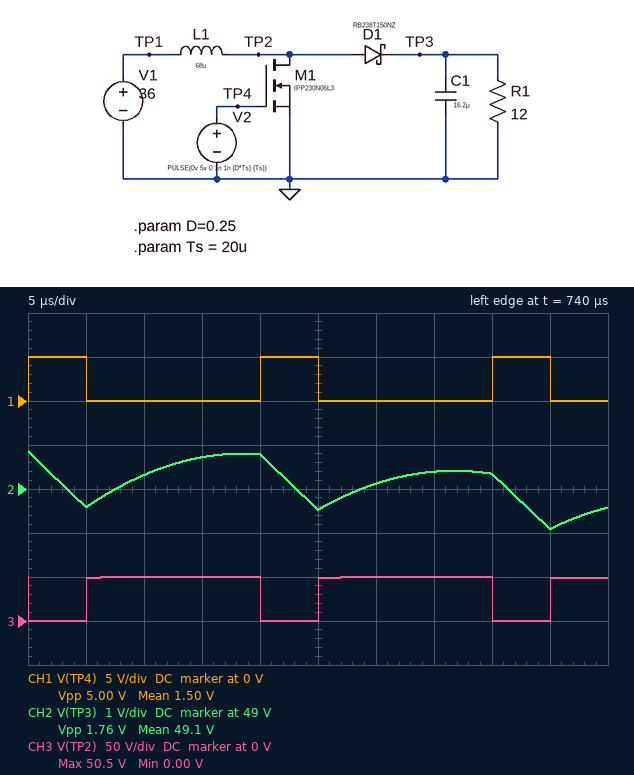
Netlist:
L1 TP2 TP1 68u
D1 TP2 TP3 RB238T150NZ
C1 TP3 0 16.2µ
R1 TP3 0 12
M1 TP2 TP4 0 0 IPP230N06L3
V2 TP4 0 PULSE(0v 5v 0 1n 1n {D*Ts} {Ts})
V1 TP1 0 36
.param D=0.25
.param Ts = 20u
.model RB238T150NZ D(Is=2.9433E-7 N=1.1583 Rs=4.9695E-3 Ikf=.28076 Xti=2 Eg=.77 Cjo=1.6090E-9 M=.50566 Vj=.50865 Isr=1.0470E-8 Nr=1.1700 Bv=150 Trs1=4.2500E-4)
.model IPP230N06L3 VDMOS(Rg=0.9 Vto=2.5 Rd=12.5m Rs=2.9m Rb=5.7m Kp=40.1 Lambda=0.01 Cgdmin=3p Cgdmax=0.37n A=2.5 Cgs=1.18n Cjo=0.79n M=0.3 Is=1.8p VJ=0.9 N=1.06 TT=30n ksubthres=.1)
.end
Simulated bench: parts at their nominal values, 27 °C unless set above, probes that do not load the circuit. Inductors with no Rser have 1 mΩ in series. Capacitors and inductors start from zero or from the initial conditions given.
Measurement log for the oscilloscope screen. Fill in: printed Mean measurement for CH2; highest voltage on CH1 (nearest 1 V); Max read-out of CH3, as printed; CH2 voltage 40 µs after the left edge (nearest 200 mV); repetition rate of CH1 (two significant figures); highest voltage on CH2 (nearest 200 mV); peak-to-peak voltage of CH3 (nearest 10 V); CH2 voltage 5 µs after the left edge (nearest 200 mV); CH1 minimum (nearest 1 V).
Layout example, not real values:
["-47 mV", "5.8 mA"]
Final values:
["49.1 V", "5 V", "50.5 V", "49.4 V", "50 kHz", "49.8 V", "50 V", "48.6 V", "0 V"]
